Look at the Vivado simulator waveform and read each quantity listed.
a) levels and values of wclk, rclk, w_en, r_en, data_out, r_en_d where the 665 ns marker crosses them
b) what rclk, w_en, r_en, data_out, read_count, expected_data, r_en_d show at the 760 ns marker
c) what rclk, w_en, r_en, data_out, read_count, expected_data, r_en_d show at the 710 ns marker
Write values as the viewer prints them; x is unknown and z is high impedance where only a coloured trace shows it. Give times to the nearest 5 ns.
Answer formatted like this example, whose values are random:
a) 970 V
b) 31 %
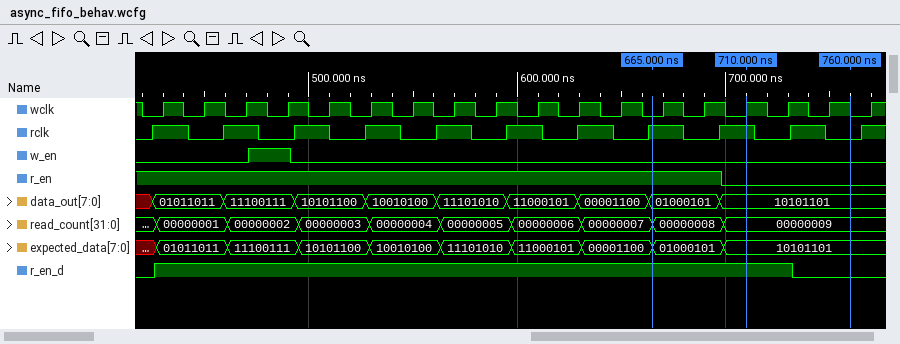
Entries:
a) wclk=0, rclk=1, w_en=0, r_en=1, data_out=01000101, r_en_d=1
b) rclk=0, w_en=0, r_en=0, data_out=10101101, read_count=00000009, expected_data=10101101, r_en_d=0
c) rclk=1, w_en=0, r_en=0, data_out=10101101, read_count=00000009, expected_data=10101101, r_en_d=1
